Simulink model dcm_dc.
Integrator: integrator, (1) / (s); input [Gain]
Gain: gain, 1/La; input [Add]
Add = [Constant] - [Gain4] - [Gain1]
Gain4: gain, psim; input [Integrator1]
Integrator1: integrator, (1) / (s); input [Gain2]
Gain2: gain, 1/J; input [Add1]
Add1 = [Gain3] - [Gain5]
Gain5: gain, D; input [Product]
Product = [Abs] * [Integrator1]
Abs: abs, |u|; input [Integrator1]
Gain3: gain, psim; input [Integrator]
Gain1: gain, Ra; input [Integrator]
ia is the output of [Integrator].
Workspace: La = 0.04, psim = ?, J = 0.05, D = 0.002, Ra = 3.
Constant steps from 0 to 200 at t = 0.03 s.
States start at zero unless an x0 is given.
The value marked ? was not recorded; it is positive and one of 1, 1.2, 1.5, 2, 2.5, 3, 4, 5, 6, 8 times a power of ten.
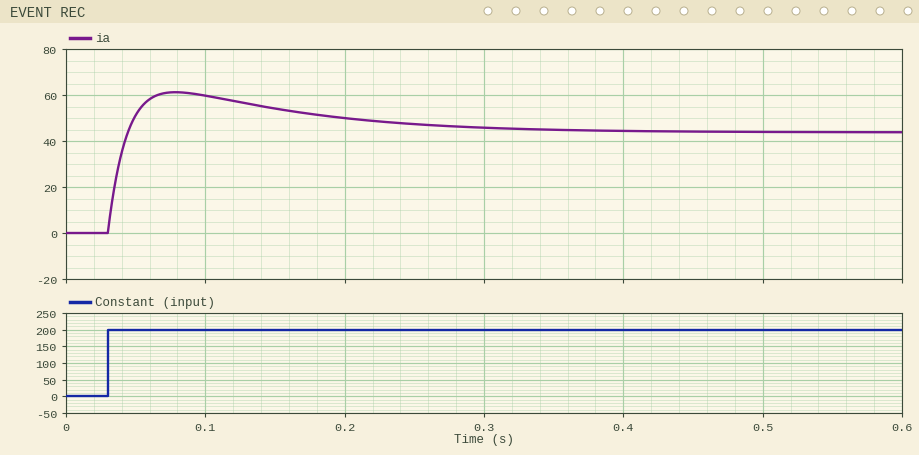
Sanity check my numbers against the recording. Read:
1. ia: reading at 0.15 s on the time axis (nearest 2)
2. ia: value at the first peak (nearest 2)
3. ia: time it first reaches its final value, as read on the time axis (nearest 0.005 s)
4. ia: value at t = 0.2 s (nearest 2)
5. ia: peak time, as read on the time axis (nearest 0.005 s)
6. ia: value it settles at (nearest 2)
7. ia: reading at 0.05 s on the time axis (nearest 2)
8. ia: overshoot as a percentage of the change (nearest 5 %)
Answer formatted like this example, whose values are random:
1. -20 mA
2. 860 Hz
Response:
1. 54
2. 62
3. 0.045 s
4. 50
5. 0.080 s
6. 44
7. 52
8. 40 %
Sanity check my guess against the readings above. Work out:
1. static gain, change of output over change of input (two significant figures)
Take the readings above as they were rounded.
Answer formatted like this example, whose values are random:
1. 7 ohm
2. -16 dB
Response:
1. 0.22
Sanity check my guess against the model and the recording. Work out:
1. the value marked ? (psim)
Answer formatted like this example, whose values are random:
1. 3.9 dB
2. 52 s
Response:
1. 0.6
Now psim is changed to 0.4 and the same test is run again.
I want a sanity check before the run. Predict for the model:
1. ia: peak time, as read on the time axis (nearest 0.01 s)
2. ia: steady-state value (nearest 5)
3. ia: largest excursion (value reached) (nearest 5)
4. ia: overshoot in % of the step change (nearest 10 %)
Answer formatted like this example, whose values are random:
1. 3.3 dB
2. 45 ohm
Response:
1. 0.09 s
2. 55
3. 65
4. 20 %
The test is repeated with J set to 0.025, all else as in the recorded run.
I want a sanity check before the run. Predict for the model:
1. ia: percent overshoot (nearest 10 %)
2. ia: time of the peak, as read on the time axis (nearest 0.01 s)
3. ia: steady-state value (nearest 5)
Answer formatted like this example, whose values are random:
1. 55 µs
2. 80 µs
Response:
1. 30 %
2. 0.07 s
3. 45
